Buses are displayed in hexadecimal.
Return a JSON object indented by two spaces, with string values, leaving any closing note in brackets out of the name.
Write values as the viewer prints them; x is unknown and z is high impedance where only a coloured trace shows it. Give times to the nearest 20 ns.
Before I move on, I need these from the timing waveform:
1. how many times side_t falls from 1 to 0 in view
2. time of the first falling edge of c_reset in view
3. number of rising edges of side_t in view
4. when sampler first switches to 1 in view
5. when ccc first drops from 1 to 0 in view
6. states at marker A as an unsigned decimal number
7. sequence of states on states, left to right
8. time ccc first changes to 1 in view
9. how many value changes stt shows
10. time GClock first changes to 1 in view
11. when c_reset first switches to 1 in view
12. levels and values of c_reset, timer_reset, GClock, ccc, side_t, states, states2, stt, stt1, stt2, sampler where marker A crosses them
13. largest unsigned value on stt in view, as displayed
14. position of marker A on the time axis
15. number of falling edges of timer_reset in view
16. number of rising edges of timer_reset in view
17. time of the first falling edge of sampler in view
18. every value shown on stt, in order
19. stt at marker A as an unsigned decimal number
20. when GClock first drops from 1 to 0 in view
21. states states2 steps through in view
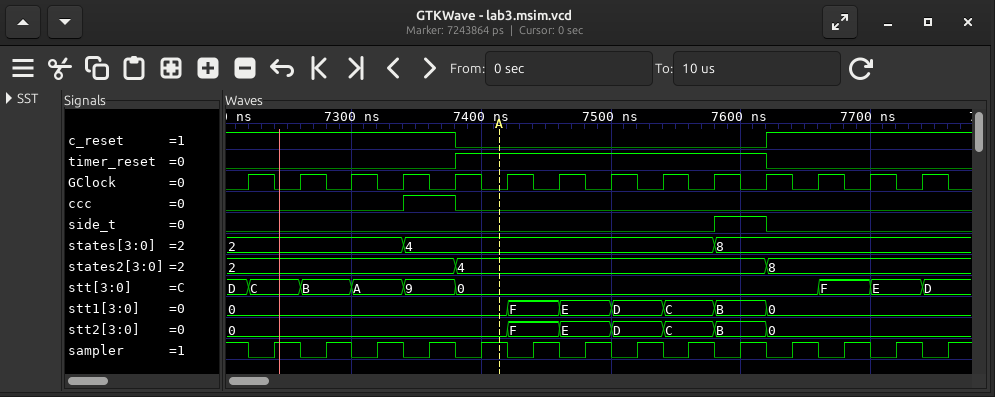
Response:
{
  "how many times side_t falls from 1 to 0 in view": "1",
  "time of the first falling edge of c_reset in view": "7380 ns",
  "number of rising edges of side_t in view": "1",
  "when sampler first switches to 1 in view": "7240 ns",
  "when ccc first drops from 1 to 0 in view": "7380 ns",
  "states at marker A as an unsigned decimal number": "4",
  "sequence of states on states, left to right": "2, 4, 8",
  "time ccc first changes to 1 in view": "7340 ns",
  "how many value changes stt shows": "8",
  "time GClock first changes to 1 in view": "7220 ns",
  "when c_reset first switches to 1 in view": "7620 ns",
  "levels and values of c_reset, timer_reset, GClock, ccc, side_t, states, states2, stt, stt1, stt2, sampler where marker A crosses them": "c_reset=0, timer_reset=1, GClock=0, ccc=0, side_t=0, states=4, states2=4, stt=0, stt1=0, stt2=0, sampler=1",
  "largest unsigned value on stt in view, as displayed": "F",
  "position of marker A on the time axis": "7420 ns",
  "number of falling edges of timer_reset in view": "1",
  "number of rising edges of timer_reset in view": "1",
  "time of the first falling edge of sampler in view": "7220 ns",
  "every value shown on stt, in order": "D, C, B, A, 9, 0, F, E, D",
  "stt at marker A as an unsigned decimal number": "0",
  "when GClock first drops from 1 to 0 in view": "7240 ns",
  "states states2 steps through in view": "2, 4, 8"
}
